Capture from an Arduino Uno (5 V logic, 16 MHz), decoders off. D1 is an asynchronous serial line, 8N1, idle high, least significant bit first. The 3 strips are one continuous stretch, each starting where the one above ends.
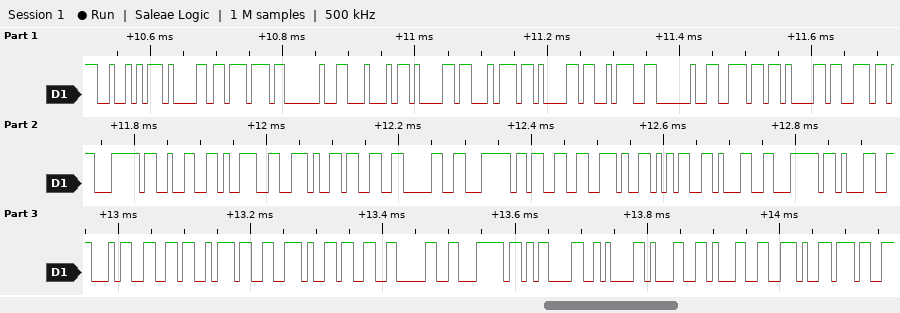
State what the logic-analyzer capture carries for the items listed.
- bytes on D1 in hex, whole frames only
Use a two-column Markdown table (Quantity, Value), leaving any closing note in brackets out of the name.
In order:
| Quantity | Value |
|---|---|
| bytes on D1 in hex, whole frames only | 0x52 0x61 0x77 0x20 0x44 0x61 0x74 0x61 0x3A 0x20 0x6E 0x61 0x6E 0x7C 0x32 0x39 0x2E 0x33 0x30 0x7C 0x33 0x2E 0x35 0x31 0x7C 0x31 0x34 0x36 0x37 0x2E 0x33 0x30 0x7C 0x0D 0x0A 0x31 0x31 0x2E 0x37 |
